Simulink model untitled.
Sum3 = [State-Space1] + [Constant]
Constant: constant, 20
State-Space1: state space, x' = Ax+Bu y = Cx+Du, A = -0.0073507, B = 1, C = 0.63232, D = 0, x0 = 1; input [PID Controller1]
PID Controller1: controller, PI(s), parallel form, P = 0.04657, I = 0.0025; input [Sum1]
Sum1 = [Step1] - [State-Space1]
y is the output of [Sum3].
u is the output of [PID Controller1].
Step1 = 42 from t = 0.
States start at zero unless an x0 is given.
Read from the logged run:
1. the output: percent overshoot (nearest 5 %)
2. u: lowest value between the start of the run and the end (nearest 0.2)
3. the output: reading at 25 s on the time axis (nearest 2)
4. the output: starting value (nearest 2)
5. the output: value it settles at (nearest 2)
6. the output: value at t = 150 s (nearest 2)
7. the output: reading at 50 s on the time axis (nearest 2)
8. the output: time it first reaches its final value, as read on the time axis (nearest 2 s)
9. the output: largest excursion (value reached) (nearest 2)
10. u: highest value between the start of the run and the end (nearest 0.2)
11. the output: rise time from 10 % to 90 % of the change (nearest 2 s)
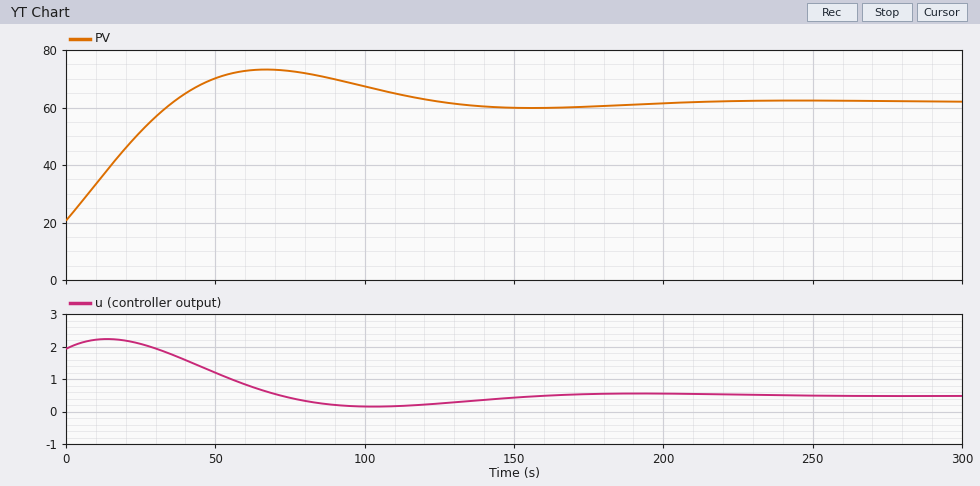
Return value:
25 %
0.2
52
20
62
60
70
36 s
74
2.2
28 s
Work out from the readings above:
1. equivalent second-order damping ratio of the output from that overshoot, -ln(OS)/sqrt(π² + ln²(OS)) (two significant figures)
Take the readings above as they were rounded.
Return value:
0.40
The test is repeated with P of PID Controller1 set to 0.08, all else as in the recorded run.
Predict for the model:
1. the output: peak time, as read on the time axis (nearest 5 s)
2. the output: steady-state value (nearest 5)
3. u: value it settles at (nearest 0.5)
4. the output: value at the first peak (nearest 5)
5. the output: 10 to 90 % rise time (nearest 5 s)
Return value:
60 s
60
0.5
70
25 s
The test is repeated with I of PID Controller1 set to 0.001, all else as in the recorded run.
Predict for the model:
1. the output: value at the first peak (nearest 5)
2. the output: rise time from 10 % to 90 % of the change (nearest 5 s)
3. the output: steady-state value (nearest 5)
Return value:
65
45 s
60
